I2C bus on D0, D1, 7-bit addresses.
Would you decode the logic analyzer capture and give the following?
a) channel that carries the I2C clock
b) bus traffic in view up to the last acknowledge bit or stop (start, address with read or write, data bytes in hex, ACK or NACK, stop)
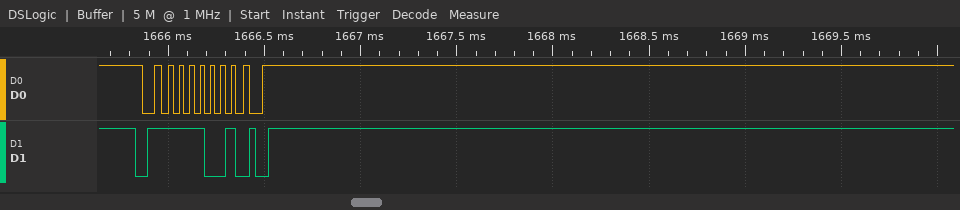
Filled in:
D0
start, address 7C read ACK, stop
